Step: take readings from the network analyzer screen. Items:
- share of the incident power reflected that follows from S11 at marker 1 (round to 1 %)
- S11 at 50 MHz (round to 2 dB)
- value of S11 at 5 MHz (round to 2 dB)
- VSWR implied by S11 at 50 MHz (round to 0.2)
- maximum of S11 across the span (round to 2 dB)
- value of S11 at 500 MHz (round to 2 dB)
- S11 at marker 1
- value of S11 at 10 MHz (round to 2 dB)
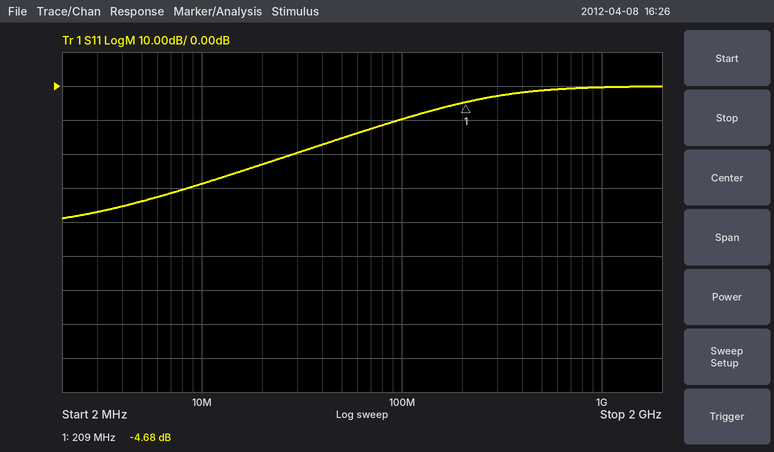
34 %
-16 dB
-34 dB
1.4
0 dB
-2 dB
-4.68 dB
-28 dB
